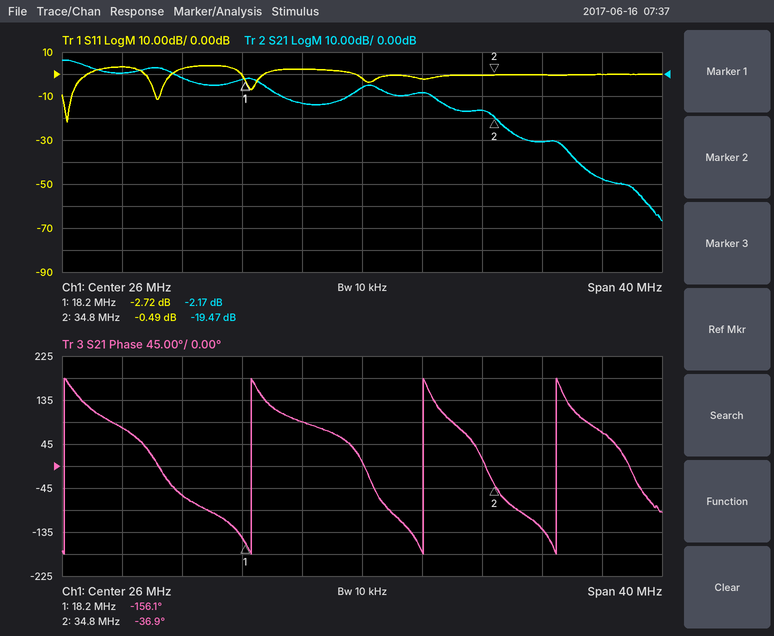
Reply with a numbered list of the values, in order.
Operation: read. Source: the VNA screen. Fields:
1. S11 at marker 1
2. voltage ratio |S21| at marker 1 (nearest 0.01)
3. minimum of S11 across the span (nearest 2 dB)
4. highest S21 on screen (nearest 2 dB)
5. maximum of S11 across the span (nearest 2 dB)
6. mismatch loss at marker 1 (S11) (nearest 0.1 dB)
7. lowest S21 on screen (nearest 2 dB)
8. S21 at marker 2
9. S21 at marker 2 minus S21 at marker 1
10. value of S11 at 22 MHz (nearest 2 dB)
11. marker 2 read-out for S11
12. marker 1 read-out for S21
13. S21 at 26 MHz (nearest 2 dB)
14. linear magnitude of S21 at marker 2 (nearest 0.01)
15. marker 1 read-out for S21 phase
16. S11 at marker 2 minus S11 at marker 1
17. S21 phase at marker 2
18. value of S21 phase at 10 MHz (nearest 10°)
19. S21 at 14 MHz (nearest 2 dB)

1. -2.72 dB
2. 0.78
3. -22 dB
4. 6 dB
5. 4 dB
6. 3.3 dB
7. -66 dB
8. -19.47 dB
9. -17.30 dB
10. 2 dB
11. -0.49 dB
12. -2.17 dB
13. -6 dB
14. 0.11
15. -156.1°
16. 2.23 dB
17. -36.9°
18. 80°
19. -2 dB
